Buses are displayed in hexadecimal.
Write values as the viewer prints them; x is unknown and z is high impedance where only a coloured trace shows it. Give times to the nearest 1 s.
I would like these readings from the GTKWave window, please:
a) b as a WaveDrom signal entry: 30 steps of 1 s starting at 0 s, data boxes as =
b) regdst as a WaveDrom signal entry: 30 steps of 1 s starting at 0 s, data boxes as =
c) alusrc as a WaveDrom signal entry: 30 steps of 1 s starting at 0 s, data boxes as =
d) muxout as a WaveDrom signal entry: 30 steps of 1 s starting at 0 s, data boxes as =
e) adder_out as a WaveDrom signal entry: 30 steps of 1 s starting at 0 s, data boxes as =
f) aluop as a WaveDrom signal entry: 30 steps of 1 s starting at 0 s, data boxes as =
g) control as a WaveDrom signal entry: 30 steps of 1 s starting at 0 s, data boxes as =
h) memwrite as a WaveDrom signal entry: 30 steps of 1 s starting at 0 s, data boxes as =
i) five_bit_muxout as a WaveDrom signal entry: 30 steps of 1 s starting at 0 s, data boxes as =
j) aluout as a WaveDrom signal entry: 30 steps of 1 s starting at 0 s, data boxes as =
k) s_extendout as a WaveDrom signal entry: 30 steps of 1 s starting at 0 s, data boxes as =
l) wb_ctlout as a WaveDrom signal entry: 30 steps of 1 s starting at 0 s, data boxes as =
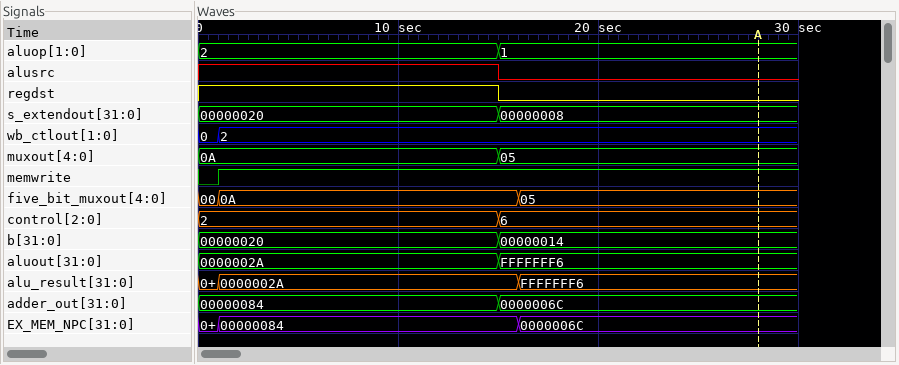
{name: 'b', wave: '=..............=..............', data: '00000020 00000014'}
{name: 'regdst', wave: '1..............0..............'}
{name: 'alusrc', wave: '1..............0..............'}
{name: 'muxout', wave: '=..............=..............', data: '0A 05'}
{name: 'adder_out', wave: '=..............=..............', data: '00000084 0000006C'}
{name: 'aluop', wave: '=..............=..............', data: '2 1'}
{name: 'control', wave: '=..............=..............', data: '2 6'}
{name: 'memwrite', wave: '01............................'}
{name: 'five_bit_muxout', wave: '==..............=.............', data: '00 0A 05'}
{name: 'aluout', wave: '=..............=..............', data: '0000002A FFFFFFF6'}
{name: 's_extendout', wave: '=..............=..............', data: '00000020 00000008'}
{name: 'wb_ctlout', wave: '==............................', data: '0 2'}
